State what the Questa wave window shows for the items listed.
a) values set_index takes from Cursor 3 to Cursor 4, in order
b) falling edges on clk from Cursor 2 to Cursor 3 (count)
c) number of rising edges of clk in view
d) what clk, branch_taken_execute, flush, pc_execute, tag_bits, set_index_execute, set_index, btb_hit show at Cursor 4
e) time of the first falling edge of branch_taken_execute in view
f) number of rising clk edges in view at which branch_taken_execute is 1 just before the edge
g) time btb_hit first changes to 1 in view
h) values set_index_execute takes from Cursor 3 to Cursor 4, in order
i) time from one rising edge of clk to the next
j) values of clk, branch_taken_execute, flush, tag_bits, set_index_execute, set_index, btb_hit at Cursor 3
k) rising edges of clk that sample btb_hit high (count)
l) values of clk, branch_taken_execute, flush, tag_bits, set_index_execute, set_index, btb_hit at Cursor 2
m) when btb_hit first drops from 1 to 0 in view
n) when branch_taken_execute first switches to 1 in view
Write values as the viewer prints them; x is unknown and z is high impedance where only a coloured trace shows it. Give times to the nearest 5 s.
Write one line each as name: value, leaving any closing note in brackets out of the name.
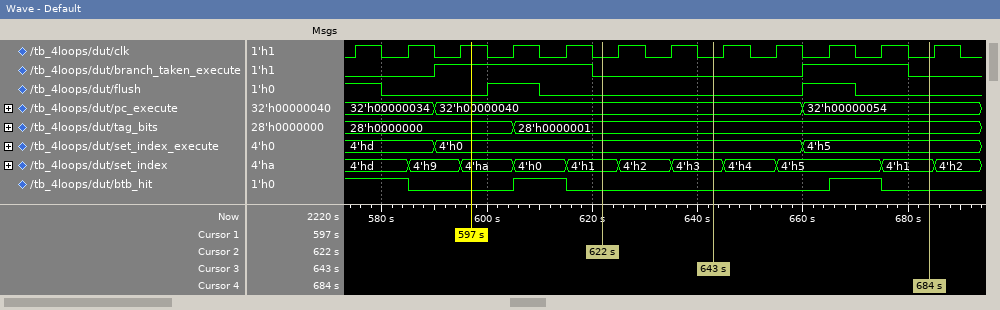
values set_index takes from Cursor 3 to Cursor 4, in order: 4'h3, 4'h4, 4'h5, 4'h1
falling edges on clk from Cursor 2 to Cursor 3: 2
number of rising edges of clk in view: 12
what clk, branch_taken_execute, flush, pc_execute, tag_bits, set_index_execute, set_index, btb_hit show at Cursor 4: clk=0, branch_taken_execute=0, flush=0, pc_execute=32'h00000054, tag_bits=28'h0000001, set_index_execute=4'h5, set_index=4'h1, btb_hit=0
time of the first falling edge of branch_taken_execute in view: 620 s
number of rising clk edges in view at which branch_taken_execute is 1 just before the edge: 5
time btb_hit first changes to 1 in view: 605 s
values set_index_execute takes from Cursor 3 to Cursor 4, in order: 4'h0, 4'h5
time from one rising edge of clk to the next: 10 s
values of clk, branch_taken_execute, flush, tag_bits, set_index_execute, set_index, btb_hit at Cursor 3: clk=0, branch_taken_execute=0, flush=0, tag_bits=28'h0000001, set_index_execute=4'h0, set_index=4'h3, btb_hit=0
rising edges of clk that sample btb_hit high: 4
values of clk, branch_taken_execute, flush, tag_bits, set_index_execute, set_index, btb_hit at Cursor 2: clk=0, branch_taken_execute=0, flush=0, tag_bits=28'h0000001, set_index_execute=4'h0, set_index=4'h1, btb_hit=0
when btb_hit first drops from 1 to 0 in view: 585 s
when branch_taken_execute first switches to 1 in view: 590 s
